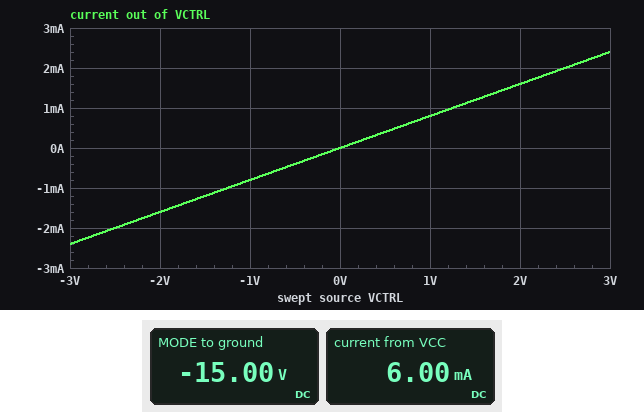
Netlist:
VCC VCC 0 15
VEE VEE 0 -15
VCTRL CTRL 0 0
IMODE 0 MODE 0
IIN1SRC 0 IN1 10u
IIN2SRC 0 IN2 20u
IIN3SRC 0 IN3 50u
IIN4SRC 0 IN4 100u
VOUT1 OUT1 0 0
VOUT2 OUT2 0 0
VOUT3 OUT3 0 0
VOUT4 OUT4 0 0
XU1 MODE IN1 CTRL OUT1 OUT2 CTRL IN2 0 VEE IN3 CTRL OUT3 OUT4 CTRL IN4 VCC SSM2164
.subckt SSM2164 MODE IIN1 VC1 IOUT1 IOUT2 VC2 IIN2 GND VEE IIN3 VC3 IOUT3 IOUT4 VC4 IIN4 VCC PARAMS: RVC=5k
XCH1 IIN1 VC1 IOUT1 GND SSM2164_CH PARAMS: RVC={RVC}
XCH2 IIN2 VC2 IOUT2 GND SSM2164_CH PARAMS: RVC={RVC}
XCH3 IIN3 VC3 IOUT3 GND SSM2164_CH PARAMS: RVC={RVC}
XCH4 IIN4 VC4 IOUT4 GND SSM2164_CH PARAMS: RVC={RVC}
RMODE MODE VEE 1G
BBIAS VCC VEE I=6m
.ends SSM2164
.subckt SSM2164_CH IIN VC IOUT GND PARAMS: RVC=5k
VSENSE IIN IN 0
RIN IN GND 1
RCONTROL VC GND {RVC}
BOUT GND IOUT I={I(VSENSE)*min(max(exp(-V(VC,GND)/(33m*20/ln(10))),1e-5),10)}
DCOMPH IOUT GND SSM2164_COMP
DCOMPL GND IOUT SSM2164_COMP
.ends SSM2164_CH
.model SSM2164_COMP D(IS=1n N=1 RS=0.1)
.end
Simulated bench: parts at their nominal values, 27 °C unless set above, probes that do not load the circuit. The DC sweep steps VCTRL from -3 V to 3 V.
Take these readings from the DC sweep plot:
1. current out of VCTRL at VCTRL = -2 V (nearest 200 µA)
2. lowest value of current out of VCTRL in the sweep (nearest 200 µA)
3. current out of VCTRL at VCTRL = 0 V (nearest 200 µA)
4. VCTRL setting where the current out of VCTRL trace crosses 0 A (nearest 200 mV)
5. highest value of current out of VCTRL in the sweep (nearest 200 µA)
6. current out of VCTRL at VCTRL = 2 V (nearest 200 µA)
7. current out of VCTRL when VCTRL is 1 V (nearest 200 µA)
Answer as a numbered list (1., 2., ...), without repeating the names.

1. -1.6 mA
2. -2.4 mA
3. 0 A
4. 0 V
5. 2.4 mA
6. 1.6 mA
7. 800 µA
